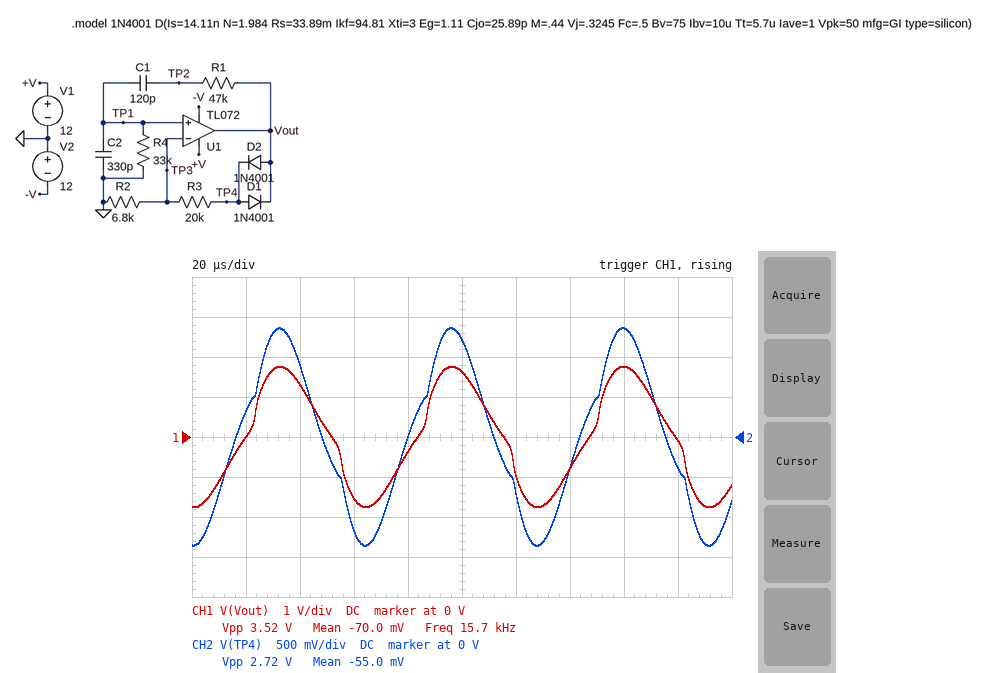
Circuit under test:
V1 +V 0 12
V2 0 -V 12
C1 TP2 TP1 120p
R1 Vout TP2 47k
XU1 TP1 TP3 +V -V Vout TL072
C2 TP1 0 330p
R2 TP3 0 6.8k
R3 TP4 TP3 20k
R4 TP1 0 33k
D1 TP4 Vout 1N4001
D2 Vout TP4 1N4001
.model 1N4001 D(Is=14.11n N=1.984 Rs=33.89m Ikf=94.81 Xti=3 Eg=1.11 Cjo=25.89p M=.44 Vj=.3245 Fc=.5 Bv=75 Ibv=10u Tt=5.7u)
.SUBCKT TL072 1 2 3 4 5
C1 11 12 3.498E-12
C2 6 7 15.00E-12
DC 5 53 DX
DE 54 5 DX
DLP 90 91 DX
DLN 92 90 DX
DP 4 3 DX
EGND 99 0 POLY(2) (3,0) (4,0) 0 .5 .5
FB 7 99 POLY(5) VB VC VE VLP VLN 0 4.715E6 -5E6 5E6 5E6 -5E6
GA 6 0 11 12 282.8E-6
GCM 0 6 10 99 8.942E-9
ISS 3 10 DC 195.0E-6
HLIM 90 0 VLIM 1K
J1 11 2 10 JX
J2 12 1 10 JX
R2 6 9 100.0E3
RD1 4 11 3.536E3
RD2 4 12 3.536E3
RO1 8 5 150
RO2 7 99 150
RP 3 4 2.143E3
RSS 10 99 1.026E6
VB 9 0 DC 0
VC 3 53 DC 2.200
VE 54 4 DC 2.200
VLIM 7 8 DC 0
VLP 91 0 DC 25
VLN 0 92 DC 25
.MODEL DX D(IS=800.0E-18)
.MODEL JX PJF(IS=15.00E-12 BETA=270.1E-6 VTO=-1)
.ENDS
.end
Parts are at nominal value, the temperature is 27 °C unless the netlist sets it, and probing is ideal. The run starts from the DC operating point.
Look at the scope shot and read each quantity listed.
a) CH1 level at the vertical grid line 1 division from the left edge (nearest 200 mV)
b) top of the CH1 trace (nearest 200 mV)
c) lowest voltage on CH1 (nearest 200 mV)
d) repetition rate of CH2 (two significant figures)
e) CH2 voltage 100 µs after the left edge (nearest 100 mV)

0 V
1.8 V
-1.8 V
16 kHz
1.2 V
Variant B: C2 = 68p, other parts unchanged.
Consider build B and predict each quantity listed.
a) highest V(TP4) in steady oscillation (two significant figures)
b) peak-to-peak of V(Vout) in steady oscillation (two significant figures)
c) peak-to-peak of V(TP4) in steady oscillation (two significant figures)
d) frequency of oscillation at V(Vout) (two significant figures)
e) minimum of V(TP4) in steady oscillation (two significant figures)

11 V
21 V
22 V
33 kHz
-11 V
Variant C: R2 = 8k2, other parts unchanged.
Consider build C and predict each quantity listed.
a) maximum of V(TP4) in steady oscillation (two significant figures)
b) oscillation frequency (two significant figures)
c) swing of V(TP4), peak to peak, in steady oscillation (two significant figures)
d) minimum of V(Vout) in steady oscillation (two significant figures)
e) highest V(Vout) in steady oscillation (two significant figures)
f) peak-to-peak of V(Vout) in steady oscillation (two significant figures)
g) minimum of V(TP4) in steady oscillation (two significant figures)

790 mV
14 kHz
1.6 V
-1.2 V
1.2 V
2.3 V
-790 mV
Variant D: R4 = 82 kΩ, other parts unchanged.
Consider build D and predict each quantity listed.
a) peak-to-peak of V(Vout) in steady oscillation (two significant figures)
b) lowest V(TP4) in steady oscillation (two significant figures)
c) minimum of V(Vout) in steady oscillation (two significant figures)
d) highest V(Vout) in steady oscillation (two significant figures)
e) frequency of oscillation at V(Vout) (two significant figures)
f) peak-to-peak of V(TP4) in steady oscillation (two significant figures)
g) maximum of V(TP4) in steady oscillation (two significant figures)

12 V
-5.7 V
-6.2 V
6.2 V
12 kHz
11 V
5.7 V
